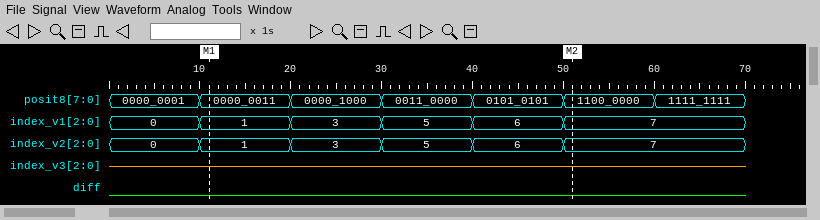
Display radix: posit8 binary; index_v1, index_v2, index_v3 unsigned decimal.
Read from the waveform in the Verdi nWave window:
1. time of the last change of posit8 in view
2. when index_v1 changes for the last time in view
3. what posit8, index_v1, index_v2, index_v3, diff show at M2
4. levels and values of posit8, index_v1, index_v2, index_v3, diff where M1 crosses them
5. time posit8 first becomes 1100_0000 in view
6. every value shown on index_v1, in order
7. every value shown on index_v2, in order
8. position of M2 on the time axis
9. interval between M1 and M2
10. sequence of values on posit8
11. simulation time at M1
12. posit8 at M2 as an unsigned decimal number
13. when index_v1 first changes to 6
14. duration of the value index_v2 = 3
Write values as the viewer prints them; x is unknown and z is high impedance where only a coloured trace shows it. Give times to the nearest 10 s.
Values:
60 s
50 s
posit8=1100_0000, index_v1=7, index_v2=7, index_v3=z, diff=0
posit8=0000_0011, index_v1=1, index_v2=1, index_v3=z, diff=0
50 s
0, 1, 3, 5, 6, 7
0, 1, 3, 5, 6, 7
50 s
40 s
0000_0001, 0000_0011, 0000_1000, 0011_0000, 0101_0101, 1100_0000, 1111_1111
10 s
192
40 s
10 s
